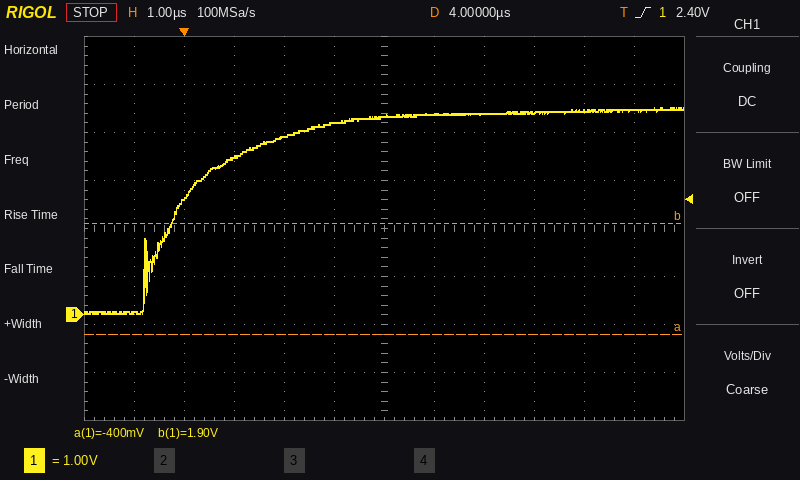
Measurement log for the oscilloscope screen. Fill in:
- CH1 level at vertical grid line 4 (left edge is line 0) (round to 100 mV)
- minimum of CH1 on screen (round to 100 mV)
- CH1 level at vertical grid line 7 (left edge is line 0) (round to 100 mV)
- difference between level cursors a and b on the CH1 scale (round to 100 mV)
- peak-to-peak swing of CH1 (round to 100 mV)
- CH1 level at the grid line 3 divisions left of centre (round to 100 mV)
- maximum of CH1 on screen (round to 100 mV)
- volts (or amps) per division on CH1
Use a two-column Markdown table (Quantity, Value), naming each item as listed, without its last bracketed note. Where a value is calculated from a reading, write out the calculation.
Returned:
| Quantity | Value |
|---|---|
| CH1 level at vertical grid line 4 (left edge is line 0) | 3.7 V |
| minimum of CH1 on screen | 0.0 V |
| CH1 level at vertical grid line 7 (left edge is line 0) | 4.2 V |
| difference between level cursors a and b on the CH1 scale | 2.3 V |
| peak-to-peak swing of CH1 | 4.3 V − (0.0 V) = 4.3 V |
| CH1 level at the grid line 3 divisions left of centre | 3.3 V |
| maximum of CH1 on screen | 4.3 V |
| volts (or amps) per division on CH1 | 1 V |
